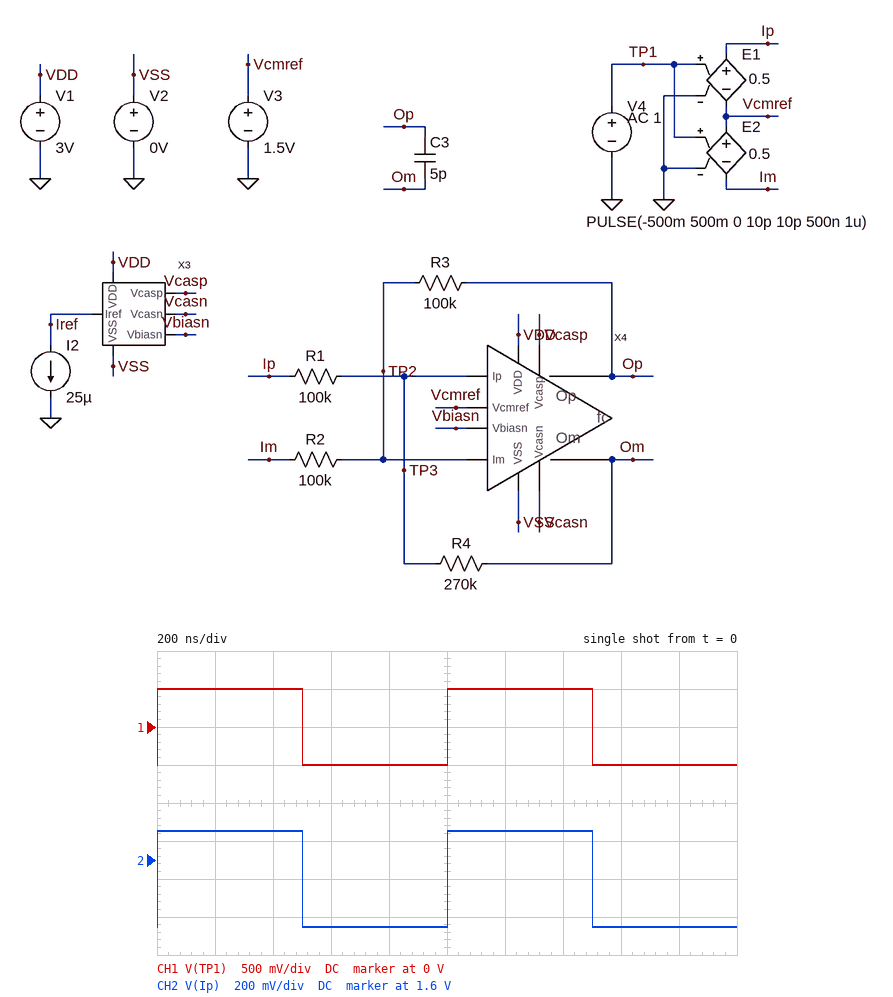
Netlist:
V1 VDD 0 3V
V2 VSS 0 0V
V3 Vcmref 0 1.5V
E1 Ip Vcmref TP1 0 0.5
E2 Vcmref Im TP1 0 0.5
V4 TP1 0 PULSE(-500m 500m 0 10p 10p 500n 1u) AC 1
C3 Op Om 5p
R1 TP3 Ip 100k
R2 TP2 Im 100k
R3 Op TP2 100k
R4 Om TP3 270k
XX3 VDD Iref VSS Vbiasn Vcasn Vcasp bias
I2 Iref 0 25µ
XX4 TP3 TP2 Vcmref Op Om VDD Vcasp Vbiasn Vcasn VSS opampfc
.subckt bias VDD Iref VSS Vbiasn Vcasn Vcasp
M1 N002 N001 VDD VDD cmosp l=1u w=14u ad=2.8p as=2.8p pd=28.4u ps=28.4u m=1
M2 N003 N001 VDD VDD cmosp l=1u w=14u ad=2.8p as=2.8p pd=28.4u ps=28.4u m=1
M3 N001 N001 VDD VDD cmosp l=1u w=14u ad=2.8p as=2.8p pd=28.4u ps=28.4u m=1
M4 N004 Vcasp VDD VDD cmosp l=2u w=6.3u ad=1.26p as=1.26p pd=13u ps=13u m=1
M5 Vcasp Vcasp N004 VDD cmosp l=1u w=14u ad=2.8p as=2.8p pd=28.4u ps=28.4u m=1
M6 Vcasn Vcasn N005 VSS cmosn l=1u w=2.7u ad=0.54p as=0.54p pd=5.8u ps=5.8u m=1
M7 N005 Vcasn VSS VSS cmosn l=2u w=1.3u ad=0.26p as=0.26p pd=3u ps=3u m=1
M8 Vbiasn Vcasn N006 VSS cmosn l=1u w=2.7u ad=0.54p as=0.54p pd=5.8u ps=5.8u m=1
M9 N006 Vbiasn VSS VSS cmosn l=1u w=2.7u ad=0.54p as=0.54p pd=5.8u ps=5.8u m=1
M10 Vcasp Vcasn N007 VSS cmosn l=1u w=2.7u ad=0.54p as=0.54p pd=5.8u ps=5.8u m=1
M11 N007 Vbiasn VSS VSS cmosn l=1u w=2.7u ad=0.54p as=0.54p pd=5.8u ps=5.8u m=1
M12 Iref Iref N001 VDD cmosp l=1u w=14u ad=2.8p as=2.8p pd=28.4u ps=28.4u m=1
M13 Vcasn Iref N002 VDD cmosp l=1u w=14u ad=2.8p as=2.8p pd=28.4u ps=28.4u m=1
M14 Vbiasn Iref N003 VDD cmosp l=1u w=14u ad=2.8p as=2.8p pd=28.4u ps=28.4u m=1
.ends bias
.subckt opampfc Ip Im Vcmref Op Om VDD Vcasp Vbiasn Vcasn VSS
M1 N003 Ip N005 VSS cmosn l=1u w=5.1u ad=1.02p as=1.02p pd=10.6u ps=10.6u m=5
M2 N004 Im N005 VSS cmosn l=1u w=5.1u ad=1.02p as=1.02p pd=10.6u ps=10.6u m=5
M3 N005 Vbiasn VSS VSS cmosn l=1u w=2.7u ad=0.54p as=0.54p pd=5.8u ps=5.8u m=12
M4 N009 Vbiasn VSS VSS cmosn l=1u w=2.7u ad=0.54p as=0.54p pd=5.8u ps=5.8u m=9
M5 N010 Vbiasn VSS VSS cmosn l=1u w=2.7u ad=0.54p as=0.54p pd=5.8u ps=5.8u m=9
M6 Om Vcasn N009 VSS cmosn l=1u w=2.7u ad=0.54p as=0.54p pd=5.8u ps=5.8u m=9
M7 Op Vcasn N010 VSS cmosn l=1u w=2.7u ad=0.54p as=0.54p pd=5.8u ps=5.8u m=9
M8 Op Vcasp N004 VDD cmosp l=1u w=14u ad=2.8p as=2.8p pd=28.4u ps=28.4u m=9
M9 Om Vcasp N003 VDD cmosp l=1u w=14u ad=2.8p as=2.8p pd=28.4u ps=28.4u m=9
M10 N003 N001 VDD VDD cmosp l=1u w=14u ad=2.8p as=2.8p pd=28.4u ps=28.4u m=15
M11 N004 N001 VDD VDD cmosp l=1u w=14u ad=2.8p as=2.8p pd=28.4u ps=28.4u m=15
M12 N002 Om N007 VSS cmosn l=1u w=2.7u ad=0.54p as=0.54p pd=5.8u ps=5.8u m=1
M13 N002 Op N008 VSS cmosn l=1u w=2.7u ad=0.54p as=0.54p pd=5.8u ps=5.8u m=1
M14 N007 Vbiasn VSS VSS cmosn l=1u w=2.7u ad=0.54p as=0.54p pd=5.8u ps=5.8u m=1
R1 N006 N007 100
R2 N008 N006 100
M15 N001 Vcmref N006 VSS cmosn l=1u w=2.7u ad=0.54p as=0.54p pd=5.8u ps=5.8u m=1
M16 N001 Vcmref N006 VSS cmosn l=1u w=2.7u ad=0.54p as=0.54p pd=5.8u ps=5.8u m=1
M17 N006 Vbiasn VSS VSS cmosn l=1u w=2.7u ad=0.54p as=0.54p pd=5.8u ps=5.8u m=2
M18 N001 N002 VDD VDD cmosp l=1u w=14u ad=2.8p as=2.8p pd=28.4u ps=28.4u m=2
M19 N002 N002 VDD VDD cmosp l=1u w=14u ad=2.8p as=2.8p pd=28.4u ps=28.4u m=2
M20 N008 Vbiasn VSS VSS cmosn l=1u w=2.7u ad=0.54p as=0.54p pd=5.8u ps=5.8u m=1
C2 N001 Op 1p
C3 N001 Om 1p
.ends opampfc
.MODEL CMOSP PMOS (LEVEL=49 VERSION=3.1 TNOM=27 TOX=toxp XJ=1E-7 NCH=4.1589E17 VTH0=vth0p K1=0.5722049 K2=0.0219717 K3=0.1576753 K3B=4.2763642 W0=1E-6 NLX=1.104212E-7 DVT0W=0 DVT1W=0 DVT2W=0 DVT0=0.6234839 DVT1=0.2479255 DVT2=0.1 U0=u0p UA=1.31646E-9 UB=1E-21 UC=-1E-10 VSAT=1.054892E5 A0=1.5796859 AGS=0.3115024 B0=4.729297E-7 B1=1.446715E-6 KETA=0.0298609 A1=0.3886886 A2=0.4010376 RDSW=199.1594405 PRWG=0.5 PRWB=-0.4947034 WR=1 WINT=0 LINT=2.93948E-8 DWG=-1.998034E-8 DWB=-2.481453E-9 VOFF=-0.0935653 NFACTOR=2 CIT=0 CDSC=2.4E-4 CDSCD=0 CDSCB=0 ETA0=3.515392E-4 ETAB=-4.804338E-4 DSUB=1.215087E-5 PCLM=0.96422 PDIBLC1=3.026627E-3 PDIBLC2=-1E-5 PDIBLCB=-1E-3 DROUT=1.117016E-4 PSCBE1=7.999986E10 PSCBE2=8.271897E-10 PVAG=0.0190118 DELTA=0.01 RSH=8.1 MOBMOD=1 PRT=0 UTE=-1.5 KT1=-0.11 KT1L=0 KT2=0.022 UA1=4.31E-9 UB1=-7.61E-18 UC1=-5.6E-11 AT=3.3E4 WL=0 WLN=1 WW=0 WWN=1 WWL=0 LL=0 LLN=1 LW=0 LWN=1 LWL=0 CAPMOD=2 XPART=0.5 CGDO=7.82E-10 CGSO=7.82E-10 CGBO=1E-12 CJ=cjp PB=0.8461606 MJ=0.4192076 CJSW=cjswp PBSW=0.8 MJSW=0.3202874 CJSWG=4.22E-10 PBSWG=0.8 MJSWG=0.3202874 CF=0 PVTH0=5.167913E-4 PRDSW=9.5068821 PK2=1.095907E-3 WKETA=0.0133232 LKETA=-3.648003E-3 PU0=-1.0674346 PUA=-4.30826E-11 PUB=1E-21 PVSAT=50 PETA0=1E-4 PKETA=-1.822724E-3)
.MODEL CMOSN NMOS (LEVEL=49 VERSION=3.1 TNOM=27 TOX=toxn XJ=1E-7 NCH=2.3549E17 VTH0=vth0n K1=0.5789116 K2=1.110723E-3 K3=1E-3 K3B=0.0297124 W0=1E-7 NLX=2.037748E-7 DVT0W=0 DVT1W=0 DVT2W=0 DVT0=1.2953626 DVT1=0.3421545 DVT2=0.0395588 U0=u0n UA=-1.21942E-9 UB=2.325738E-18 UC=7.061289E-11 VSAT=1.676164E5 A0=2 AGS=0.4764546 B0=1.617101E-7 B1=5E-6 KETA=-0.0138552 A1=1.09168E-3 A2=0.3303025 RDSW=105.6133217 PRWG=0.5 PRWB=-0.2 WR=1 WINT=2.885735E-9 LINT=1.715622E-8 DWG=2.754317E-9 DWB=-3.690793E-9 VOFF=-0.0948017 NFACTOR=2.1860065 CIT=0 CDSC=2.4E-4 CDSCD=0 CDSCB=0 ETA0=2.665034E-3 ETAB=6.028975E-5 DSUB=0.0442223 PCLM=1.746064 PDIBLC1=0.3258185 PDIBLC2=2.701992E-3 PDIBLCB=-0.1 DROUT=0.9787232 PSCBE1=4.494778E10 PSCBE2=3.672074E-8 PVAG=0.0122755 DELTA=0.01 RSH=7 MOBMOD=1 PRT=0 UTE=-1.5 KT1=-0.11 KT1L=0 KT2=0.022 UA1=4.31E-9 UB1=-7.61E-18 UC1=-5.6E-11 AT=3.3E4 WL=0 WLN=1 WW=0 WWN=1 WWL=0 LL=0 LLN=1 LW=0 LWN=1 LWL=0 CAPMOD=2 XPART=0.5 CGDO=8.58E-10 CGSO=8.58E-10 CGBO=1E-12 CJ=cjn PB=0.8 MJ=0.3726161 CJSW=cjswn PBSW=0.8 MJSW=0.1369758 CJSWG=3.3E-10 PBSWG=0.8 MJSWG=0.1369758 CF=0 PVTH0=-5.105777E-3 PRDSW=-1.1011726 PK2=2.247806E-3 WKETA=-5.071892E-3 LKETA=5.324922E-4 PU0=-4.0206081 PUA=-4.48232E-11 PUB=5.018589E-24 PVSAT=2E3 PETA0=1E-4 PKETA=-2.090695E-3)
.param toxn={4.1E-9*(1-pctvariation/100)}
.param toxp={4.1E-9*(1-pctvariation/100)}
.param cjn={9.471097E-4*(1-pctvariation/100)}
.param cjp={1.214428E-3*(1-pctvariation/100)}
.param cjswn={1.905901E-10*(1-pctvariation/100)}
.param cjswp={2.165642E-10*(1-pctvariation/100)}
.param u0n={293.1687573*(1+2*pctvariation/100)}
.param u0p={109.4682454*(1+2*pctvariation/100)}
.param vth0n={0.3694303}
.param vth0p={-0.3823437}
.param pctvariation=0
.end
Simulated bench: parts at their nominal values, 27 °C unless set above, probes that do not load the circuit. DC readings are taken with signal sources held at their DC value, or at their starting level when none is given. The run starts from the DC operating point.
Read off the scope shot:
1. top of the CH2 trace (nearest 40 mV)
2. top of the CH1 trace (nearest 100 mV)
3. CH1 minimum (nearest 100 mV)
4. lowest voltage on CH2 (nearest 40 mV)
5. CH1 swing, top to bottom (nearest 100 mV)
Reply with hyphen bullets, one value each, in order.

- 1.76 V
- 500 mV
- -500 mV
- 1.24 V
- 1.0 V
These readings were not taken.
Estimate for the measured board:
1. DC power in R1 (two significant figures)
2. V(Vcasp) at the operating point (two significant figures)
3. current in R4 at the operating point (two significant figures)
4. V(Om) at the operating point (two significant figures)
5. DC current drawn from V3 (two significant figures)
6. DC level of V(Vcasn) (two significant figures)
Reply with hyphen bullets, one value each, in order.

- 100 nW
- 2.0 V
- 1.0 µA
- 1.6 V
- 2.9 µA
- 1.1 V
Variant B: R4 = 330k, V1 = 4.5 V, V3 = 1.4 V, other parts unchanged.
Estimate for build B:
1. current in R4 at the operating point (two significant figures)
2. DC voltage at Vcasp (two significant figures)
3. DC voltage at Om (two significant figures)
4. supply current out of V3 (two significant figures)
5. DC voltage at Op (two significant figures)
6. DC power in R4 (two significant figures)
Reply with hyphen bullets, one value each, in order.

- 870 nA
- 3.5 V
- 1.5 V
- 3.2 µA
- 830 mV
- 250 nW
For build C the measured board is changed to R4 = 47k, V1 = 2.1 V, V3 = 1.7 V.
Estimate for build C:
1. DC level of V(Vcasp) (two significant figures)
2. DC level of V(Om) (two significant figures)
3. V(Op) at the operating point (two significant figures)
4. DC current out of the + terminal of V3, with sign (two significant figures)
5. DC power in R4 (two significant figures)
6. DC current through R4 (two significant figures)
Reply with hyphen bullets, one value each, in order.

- 1.1 V
- 1.8 V
- 1.5 V
- -200 nA
- 290 nW
- 2.5 µA
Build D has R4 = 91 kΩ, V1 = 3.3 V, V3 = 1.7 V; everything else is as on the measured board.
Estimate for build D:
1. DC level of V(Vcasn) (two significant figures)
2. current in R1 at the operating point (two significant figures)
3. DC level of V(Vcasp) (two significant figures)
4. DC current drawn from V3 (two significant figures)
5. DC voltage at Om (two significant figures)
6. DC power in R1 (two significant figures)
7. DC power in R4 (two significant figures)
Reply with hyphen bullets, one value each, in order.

- 1.1 V
- 2.0 µA
- 2.3 V
- 1.0 µA
- 1.8 V
- 390 nW
- 350 nW
